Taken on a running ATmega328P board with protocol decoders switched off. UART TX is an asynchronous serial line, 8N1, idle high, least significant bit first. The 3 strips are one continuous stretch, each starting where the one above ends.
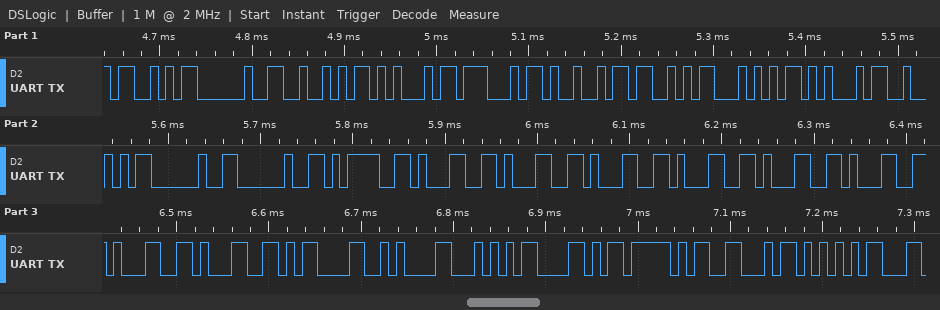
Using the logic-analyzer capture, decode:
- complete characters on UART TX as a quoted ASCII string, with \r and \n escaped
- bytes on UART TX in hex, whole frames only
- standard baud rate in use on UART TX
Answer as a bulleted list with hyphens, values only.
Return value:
- "S REGISTER  =11111111\r\nTX_FU"
- 53 20 52 45 47 49 53 54 45 52 20 20 3D 31 31 31 31 31 31 31 31 0D 0A 54 58 5F 46 55
- 115200 baud
